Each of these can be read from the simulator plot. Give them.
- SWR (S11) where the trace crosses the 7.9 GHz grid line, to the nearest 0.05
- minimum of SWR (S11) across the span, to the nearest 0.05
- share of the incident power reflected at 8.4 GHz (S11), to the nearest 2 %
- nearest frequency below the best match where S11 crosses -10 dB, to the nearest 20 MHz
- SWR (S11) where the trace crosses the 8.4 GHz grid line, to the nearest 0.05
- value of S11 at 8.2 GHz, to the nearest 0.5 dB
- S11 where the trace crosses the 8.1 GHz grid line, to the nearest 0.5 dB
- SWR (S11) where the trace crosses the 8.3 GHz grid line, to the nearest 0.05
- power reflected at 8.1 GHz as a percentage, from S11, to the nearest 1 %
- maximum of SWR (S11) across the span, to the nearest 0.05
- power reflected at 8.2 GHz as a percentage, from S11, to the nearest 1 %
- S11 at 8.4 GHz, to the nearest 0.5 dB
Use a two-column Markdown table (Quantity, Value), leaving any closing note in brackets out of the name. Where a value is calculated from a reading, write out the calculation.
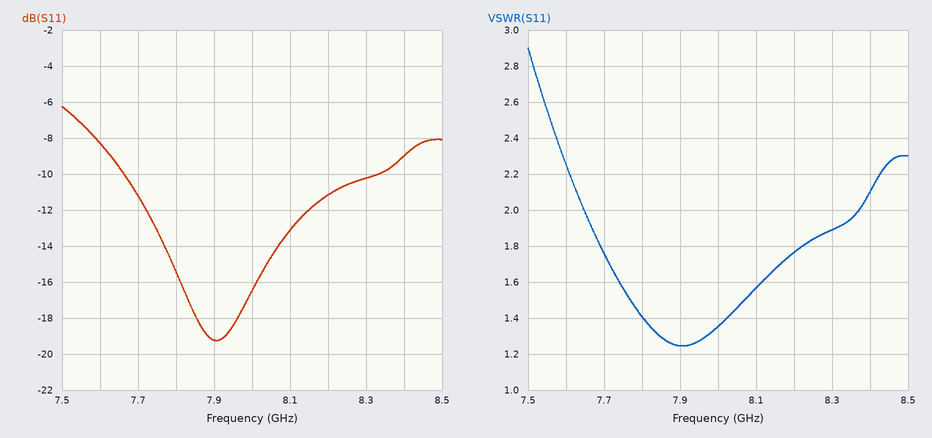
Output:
| Quantity | Value |
|---|---|
| SWR (S11) where the trace crosses the 7.9 GHz grid line, to the nearest 0.05 | 1.25 |
| minimum of SWR (S11) across the span, to the nearest 0.05 | 1.25 |
| share of the incident power reflected at 8.4 GHz (S11), to the nearest 2 % | 10^(-9/10) ≈ 12.6 %, so 12 % to the nearest 2 % |
| nearest frequency below the best match where S11 crosses -10 dB, to the nearest 20 MHz | 7.66 GHz |
| SWR (S11) where the trace crosses the 8.4 GHz grid line, to the nearest 0.05 | 2.10 |
| value of S11 at 8.2 GHz, to the nearest 0.5 dB | -11.0 dB |
| S11 where the trace crosses the 8.1 GHz grid line, to the nearest 0.5 dB | -13.0 dB |
| SWR (S11) where the trace crosses the 8.3 GHz grid line, to the nearest 0.05 | 1.90 |
| power reflected at 8.1 GHz as a percentage, from S11, to the nearest 1 % | 10^(-13/10) ≈ 5 % |
| maximum of SWR (S11) across the span, to the nearest 0.05 | 2.90 |
| power reflected at 8.2 GHz as a percentage, from S11, to the nearest 1 % | 10^(-11/10) ≈ 8 % |
| S11 at 8.4 GHz, to the nearest 0.5 dB | -9.0 dB |
